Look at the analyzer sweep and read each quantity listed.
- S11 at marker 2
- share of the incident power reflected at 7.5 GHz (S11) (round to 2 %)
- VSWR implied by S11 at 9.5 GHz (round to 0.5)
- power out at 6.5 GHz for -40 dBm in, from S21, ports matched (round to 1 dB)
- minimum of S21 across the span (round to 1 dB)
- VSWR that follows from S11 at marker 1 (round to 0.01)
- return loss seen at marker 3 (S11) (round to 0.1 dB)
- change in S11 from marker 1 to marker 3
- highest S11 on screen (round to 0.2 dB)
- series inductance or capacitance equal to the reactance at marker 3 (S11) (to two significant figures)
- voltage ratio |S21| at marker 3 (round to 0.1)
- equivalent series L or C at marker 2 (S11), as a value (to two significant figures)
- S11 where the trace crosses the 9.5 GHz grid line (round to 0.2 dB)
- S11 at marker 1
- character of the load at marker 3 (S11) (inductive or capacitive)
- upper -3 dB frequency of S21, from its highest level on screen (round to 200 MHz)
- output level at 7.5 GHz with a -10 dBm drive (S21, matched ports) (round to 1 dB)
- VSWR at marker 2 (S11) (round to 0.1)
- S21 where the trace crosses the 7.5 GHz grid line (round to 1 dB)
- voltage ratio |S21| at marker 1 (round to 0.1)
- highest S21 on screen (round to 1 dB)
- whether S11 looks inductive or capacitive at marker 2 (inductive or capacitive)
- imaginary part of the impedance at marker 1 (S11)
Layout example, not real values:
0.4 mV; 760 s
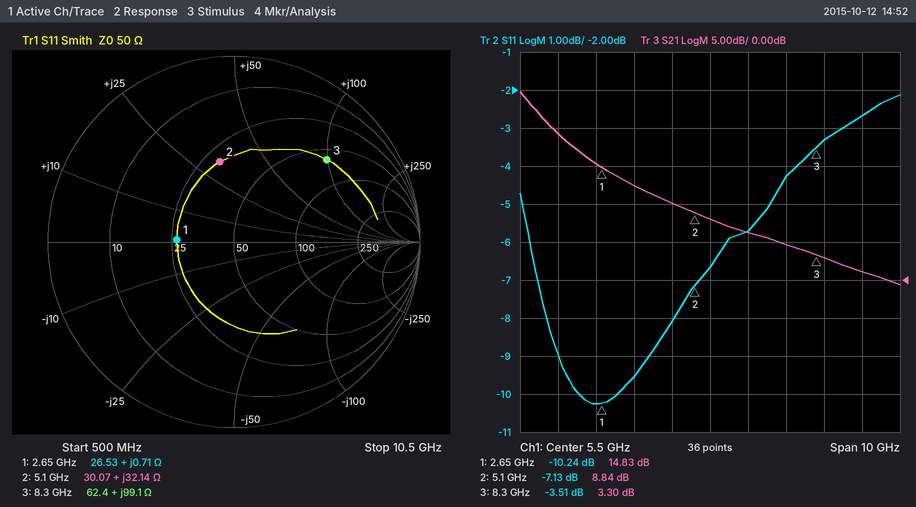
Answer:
-7.13 dB; 38 %; 6.5; -34 dBm; -1 dB; 1.89; 3.5 dB; 6.73 dB; -2.2 dB; 1.9 nH; 1.5; 1.0 nH; -2.6 dB; -10.24 dB; inductive; 1.0 GHz; -5 dBm; 2.6; 5 dB; 5.5; 25 dB; inductive; +0.71 Ω
